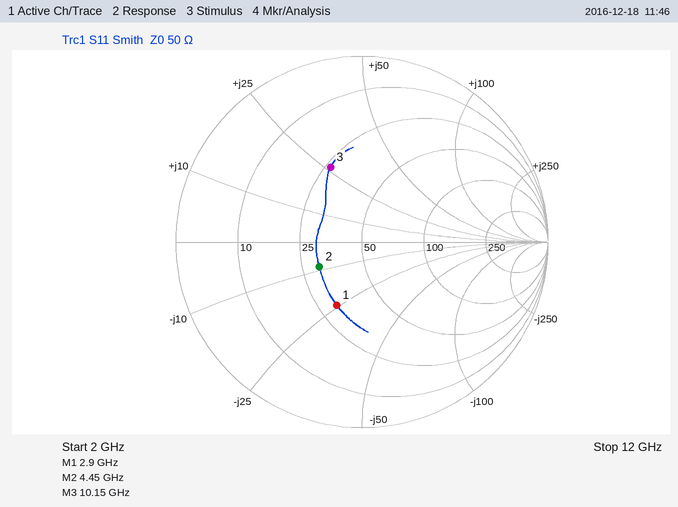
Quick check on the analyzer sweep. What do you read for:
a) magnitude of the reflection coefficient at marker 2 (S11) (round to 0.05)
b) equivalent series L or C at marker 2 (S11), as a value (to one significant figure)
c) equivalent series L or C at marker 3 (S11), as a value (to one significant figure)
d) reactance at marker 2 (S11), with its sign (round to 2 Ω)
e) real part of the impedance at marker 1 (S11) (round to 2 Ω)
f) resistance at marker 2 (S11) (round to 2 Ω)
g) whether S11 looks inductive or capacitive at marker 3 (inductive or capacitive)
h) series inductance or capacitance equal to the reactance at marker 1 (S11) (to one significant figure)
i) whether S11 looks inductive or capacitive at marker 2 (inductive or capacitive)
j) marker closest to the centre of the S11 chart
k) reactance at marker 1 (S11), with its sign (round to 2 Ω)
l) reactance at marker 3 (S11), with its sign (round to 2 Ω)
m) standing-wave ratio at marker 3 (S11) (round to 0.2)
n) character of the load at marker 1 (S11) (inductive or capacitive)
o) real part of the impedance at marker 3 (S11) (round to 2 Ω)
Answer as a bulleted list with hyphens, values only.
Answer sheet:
- 0.25
- 4 pF
- 400 pH
- -8 Ω
- 30 Ω
- 30 Ω
- inductive
- 2 pF
- capacitive
- marker 2
- -24 Ω
- +26 Ω
- 2.6
- capacitive
- 26 Ω
